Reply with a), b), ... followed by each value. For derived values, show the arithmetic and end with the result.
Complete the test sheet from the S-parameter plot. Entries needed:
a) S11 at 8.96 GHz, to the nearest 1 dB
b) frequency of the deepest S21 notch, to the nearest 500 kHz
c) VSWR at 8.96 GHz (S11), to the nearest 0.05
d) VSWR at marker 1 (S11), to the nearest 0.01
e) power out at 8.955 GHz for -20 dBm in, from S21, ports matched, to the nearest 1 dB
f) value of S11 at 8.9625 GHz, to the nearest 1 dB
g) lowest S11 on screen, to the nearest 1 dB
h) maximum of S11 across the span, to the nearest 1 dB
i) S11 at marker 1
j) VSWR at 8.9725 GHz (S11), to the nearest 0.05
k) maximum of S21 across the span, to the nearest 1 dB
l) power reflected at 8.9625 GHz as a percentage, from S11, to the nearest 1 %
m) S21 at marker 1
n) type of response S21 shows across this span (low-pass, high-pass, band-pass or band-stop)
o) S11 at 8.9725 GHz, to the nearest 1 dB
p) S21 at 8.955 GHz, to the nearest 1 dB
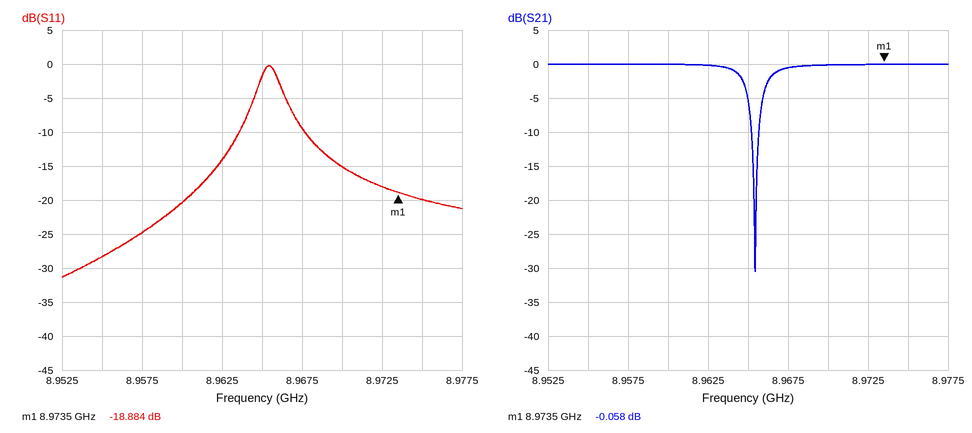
a) -20 dB
b) 8.9655 GHz
c) |Γ| = 10^(-20/20) = 0.1000; VSWR = (1 + 0.1000)/(1 − 0.1000) ≈ 1.22, so 1.20 to the nearest 0.05
d) (1 + 0.1137)/(1 − 0.1137) ≈ 1.26
e) -20 dBm + (0 dB) = -20 dBm
f) -14 dB
g) -31 dB
h) 0 dB
i) -18.884 dB
j) |Γ| = 10^(-18/20) = 0.1259; VSWR = (1 + 0.1259)/(1 − 0.1259) ≈ 1.29, so 1.30 to the nearest 0.05
k) 0 dB
l) 10^(-14/10) ≈ 4 %
m) -0.058 dB
n) band-stop
o) -18 dB
p) 0 dB
